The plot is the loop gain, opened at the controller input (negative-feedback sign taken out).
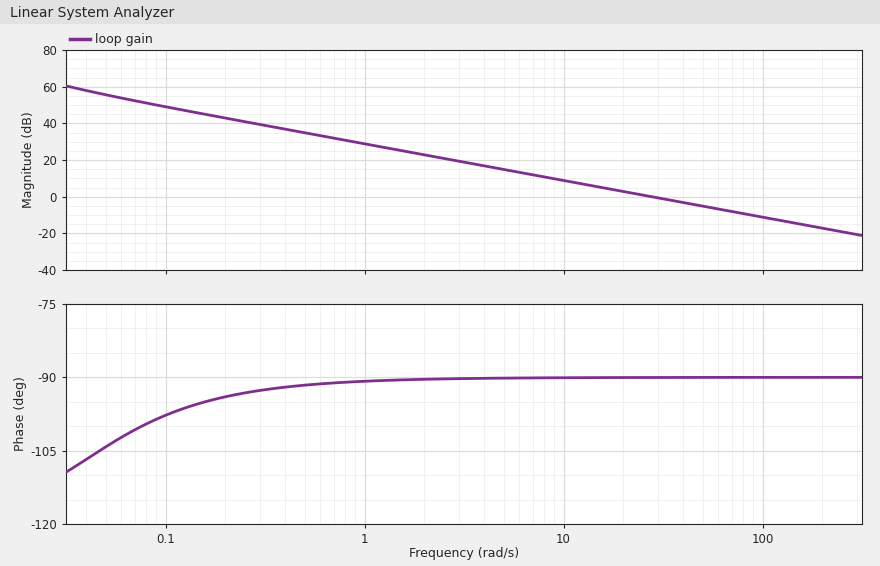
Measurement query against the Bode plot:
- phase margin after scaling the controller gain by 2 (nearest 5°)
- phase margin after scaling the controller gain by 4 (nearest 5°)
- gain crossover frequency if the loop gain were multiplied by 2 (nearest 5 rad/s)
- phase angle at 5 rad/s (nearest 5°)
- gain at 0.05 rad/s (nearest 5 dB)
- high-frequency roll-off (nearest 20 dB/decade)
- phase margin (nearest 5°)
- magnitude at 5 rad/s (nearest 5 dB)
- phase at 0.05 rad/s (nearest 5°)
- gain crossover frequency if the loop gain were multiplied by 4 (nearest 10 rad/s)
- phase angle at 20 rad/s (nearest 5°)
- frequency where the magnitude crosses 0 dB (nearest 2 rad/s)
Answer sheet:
90°
90°
55 rad/s
-90°
55 dB
-20 dB/decade
90°
15 dB
-105°
110 rad/s
-90°
28 rad/s
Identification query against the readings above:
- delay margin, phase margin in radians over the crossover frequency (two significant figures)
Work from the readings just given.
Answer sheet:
0.056 s
